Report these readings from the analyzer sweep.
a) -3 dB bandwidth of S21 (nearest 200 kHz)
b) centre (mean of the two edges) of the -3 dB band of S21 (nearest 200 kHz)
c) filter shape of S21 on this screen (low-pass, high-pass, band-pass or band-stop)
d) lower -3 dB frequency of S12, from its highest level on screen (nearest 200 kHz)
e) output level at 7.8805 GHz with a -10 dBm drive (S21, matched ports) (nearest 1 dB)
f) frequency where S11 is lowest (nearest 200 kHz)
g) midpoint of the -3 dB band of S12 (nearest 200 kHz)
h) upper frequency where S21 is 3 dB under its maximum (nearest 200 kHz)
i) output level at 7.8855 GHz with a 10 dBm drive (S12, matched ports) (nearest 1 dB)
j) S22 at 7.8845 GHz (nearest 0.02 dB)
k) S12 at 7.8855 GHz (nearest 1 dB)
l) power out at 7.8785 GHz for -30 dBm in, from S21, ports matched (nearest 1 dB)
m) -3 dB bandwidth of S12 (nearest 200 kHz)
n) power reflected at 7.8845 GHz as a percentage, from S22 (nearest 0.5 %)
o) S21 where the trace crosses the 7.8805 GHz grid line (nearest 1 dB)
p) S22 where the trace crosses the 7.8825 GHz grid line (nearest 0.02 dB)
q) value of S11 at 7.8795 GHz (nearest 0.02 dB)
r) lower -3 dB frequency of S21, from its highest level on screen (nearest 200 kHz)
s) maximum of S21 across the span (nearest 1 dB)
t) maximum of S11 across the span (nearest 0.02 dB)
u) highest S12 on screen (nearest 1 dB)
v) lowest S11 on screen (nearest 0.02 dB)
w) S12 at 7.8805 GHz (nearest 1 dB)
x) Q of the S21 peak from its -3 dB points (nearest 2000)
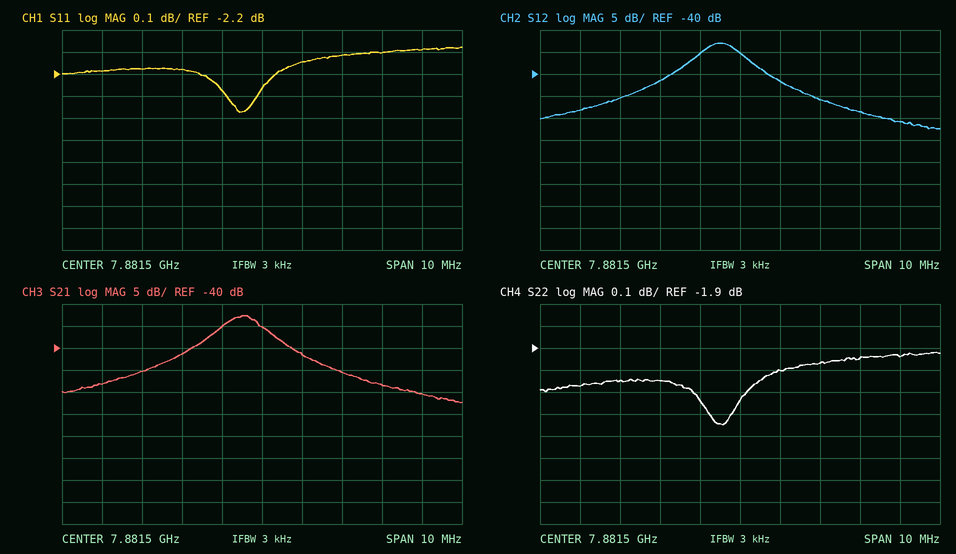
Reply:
1.2 MHz
7.8810 GHz
band-pass
7.8804 GHz
-45 dBm
7.8810 GHz
7.8810 GHz
7.8816 GHz
-41 dBm
-1.94 dB
-51 dB
-75 dBm
1.2 MHz
64.0 %
-35 dB
-2.00 dB
-2.18 dB
7.8804 GHz
-33 dB
-2.08 dB
-33 dB
-2.38 dB
-35 dB
6000
